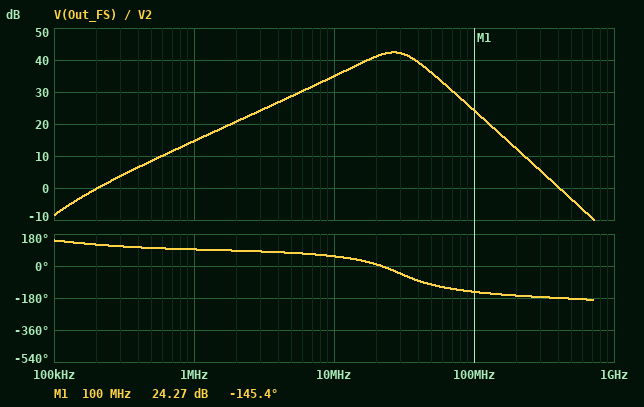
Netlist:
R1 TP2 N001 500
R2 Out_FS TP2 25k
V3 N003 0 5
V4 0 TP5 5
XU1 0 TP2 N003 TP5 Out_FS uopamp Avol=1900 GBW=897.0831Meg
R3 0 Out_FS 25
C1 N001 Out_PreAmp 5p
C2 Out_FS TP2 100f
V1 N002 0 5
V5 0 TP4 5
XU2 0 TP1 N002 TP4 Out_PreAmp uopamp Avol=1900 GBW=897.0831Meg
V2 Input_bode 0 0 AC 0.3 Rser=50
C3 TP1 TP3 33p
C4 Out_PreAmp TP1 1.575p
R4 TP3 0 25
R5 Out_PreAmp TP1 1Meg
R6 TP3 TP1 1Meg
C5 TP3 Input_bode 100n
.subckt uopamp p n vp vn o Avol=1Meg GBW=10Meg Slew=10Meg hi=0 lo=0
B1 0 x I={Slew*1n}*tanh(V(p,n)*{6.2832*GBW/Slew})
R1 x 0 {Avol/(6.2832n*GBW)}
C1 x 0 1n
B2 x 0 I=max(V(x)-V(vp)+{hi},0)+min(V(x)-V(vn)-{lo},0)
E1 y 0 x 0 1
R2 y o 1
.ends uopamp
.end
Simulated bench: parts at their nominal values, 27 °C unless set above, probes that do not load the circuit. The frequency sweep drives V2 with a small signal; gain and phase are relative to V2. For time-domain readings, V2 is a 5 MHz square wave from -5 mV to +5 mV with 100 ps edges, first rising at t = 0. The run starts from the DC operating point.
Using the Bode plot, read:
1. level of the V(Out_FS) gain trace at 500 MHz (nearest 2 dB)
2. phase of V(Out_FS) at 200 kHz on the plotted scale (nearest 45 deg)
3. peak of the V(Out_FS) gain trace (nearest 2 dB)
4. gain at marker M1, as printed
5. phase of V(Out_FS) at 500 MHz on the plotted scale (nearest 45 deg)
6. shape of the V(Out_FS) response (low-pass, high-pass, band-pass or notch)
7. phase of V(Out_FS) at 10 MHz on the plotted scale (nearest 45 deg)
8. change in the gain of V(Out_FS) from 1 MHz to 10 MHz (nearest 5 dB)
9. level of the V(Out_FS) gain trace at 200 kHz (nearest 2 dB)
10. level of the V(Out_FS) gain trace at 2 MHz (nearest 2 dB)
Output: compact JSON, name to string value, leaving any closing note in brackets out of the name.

{"level of the V(Out_FS) gain trace at 500 MHz": "-4 dB", "phase of V(Out_FS) at 200 kHz on the plotted scale": "135 deg", "peak of the V(Out_FS) gain trace": "42 dB", "gain at marker M1, as printed": "24.27 dB", "phase of V(Out_FS) at 500 MHz on the plotted scale": "-180 deg", "shape of the V(Out_FS) response": "band-pass", "phase of V(Out_FS) at 10 MHz on the plotted scale": "45 deg", "change in the gain of V(Out_FS) from 1 MHz to 10 MHz": "20 dB", "level of the V(Out_FS) gain trace at 200 kHz": "0 dB", "level of the V(Out_FS) gain trace at 2 MHz": "20 dB"}
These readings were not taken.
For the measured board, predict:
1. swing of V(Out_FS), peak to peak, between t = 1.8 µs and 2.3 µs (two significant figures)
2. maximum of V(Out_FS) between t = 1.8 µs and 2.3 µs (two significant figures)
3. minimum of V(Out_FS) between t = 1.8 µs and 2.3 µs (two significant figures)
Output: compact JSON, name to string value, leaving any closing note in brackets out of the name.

{"swing of V(Out_FS), peak to peak, between t = 1.8 µs and 2.3 µs": "620 mV", "maximum of V(Out_FS) between t = 1.8 µs and 2.3 µs": "310 mV", "minimum of V(Out_FS) between t = 1.8 µs and 2.3 µs": "-310 mV"}
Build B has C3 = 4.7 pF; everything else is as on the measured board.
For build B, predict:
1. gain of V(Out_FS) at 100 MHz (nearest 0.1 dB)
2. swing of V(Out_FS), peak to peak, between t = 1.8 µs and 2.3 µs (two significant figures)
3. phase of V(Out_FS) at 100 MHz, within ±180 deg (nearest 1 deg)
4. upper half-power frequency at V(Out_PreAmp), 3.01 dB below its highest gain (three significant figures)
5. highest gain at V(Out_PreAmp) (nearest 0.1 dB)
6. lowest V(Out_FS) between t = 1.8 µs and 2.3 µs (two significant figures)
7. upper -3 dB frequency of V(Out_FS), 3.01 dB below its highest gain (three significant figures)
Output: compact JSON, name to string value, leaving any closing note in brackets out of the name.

{"gain of V(Out_FS) at 100 MHz": "15.8 dB", "swing of V(Out_FS), peak to peak, between t = 1.8 µs and 2.3 µs": "200 mV", "phase of V(Out_FS) at 100 MHz, within ±180 deg": "-101 deg", "upper half-power frequency at V(Out_PreAmp), 3.01 dB below its highest gain": "208 MHz", "highest gain at V(Out_PreAmp)": "-0.1 dB", "lowest V(Out_FS) between t = 1.8 µs and 2.3 µs": "-100 mV", "upper -3 dB frequency of V(Out_FS), 3.01 dB below its highest gain": "45.4 MHz"}
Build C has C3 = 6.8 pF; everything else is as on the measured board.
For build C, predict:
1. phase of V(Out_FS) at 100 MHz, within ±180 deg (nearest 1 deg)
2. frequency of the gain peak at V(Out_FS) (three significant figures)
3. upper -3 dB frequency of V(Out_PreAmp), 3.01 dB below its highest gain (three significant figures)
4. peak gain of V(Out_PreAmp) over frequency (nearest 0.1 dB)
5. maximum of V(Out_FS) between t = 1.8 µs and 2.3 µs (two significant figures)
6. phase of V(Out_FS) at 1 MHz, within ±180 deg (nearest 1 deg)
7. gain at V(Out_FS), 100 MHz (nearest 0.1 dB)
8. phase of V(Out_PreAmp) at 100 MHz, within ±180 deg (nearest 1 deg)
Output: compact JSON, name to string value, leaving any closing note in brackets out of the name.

{"phase of V(Out_FS) at 100 MHz, within ±180 deg": "-108 deg", "frequency of the gain peak at V(Out_FS)": "28.8 MHz", "upper -3 dB frequency of V(Out_PreAmp), 3.01 dB below its highest gain": "154 MHz", "peak gain of V(Out_PreAmp) over frequency": "3.1 dB", "maximum of V(Out_FS) between t = 1.8 µs and 2.3 µs": "130 mV", "phase of V(Out_FS) at 1 MHz, within ±180 deg": "93 deg", "gain at V(Out_FS), 100 MHz": "18.4 dB", "phase of V(Out_PreAmp) at 100 MHz, within ±180 deg": "146 deg"}
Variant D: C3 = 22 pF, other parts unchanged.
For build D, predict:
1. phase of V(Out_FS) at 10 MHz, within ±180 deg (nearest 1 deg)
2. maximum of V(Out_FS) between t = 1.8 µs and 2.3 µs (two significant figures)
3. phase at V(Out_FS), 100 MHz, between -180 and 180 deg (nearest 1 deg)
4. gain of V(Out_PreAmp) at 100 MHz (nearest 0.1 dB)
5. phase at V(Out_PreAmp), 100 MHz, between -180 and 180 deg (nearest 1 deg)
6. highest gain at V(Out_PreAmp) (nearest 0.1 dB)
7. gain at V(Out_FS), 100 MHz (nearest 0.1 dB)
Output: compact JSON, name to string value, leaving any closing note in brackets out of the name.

{"phase of V(Out_FS) at 10 MHz, within ±180 deg": "59 deg", "maximum of V(Out_FS) between t = 1.8 µs and 2.3 µs": "250 mV", "phase at V(Out_FS), 100 MHz, between -180 and 180 deg": "-137 deg", "gain of V(Out_PreAmp) at 100 MHz": "6.8 dB", "phase at V(Out_PreAmp), 100 MHz, between -180 and 180 deg": "117 deg", "highest gain at V(Out_PreAmp)": "13.3 dB", "gain at V(Out_FS), 100 MHz": "23.6 dB"}
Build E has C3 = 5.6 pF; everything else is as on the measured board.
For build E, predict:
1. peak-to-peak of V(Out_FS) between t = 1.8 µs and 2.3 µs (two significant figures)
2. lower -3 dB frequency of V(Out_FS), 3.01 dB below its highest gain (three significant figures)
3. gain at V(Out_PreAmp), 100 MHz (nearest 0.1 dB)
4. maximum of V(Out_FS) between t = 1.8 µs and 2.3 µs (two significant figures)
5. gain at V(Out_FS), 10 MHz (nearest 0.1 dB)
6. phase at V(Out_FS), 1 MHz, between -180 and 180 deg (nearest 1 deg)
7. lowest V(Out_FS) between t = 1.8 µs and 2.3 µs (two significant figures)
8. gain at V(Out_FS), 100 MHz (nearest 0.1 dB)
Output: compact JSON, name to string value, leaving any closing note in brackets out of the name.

{"peak-to-peak of V(Out_FS) between t = 1.8 µs and 2.3 µs": "230 mV", "lower -3 dB frequency of V(Out_FS), 3.01 dB below its highest gain": "18.2 MHz", "gain at V(Out_PreAmp), 100 MHz": "0.3 dB", "maximum of V(Out_FS) between t = 1.8 µs and 2.3 µs": "110 mV", "gain at V(Out_FS), 10 MHz": "19.9 dB", "phase at V(Out_FS), 1 MHz, between -180 and 180 deg": "93 deg", "lowest V(Out_FS) between t = 1.8 µs and 2.3 µs": "-110 mV", "gain at V(Out_FS), 100 MHz": "17.1 dB"}
